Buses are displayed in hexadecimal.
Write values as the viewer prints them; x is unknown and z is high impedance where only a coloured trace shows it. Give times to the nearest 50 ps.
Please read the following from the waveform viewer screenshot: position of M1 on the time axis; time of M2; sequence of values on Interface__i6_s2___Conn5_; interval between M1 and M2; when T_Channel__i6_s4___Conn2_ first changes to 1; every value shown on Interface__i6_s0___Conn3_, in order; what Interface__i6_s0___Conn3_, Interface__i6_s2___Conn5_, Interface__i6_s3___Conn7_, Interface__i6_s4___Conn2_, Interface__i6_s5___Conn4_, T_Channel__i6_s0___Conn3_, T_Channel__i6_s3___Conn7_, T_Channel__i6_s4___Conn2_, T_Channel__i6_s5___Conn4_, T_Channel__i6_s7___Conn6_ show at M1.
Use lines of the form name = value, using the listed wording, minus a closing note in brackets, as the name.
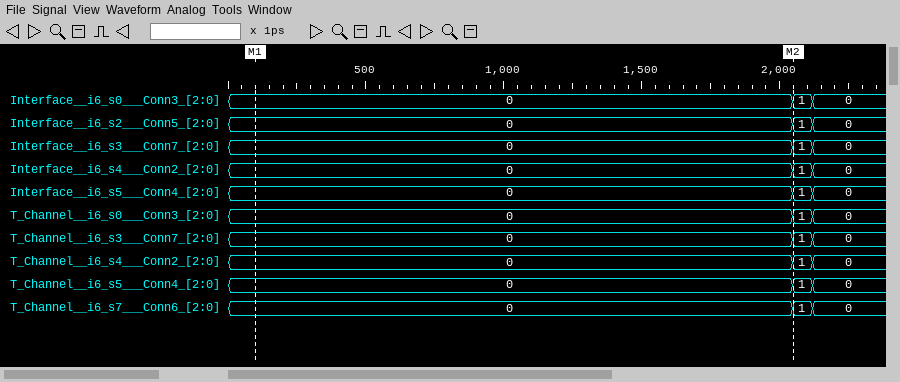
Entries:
position of M1 on the time axis = 100 ps
time of M2 = 2050 ps
sequence of values on Interface__i6_s2___Conn5_ = 0, 1, 0
interval between M1 and M2 = 1950 ps
when T_Channel__i6_s4___Conn2_ first changes to 1 = 2050 ps
every value shown on Interface__i6_s0___Conn3_, in order = 0, 1, 0
what Interface__i6_s0___Conn3_, Interface__i6_s2___Conn5_, Interface__i6_s3___Conn7_, Interface__i6_s4___Conn2_, Interface__i6_s5___Conn4_, T_Channel__i6_s0___Conn3_, T_Channel__i6_s3___Conn7_, T_Channel__i6_s4___Conn2_, T_Channel__i6_s5___Conn4_, T_Channel__i6_s7___Conn6_ show at M1 = Interface__i6_s0___Conn3_=0, Interface__i6_s2___Conn5_=0, Interface__i6_s3___Conn7_=0, Interface__i6_s4___Conn2_=0, Interface__i6_s5___Conn4_=0, T_Channel__i6_s0___Conn3_=0, T_Channel__i6_s3___Conn7_=0, T_Channel__i6_s4___Conn2_=0, T_Channel__i6_s5___Conn4_=0, T_Channel__i6_s7___Conn6_=0
